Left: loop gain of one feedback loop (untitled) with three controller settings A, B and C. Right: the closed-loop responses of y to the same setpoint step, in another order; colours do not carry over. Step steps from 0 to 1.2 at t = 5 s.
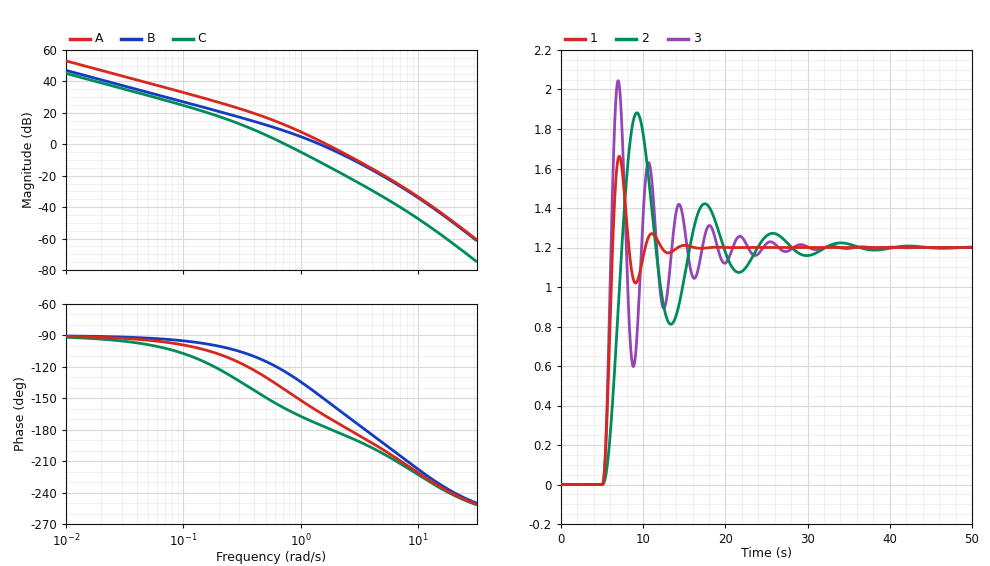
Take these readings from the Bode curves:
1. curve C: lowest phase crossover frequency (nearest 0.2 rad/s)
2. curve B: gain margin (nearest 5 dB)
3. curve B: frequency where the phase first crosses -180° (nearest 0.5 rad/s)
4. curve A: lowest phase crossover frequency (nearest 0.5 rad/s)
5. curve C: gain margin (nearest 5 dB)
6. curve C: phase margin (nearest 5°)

1.8 rad/s
15 dB
3.5 rad/s
2.5 rad/s
15 dB
20°
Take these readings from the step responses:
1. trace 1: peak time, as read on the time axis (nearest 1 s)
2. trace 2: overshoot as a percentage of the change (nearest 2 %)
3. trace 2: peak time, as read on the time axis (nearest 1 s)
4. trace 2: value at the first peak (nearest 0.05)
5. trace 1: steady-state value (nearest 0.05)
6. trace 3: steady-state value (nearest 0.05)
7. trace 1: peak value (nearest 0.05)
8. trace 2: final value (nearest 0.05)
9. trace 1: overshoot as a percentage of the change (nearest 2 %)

7 s
56 %
9 s
1.90
1.20
1.20
1.65
1.20
38 %
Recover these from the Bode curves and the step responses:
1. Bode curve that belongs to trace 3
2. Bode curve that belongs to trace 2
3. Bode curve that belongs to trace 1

A
C
B
